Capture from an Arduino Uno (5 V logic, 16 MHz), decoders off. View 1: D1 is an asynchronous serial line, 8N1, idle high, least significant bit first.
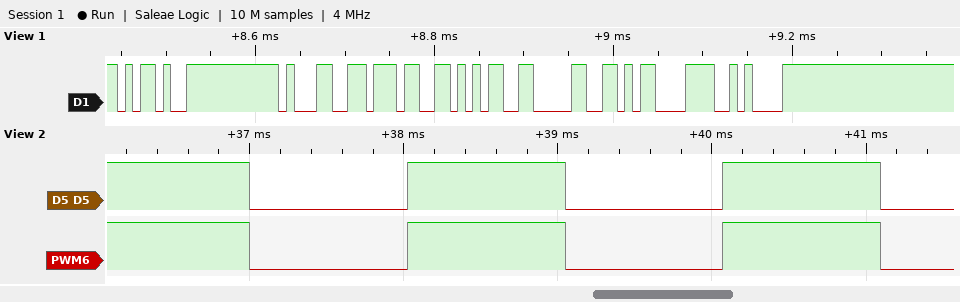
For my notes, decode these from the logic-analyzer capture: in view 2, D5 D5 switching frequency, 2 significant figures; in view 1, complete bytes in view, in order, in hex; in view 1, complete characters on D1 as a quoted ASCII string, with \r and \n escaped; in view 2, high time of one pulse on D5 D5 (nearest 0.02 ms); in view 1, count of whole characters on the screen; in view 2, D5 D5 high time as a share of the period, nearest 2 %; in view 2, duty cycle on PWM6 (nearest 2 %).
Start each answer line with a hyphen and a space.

- 490 Hz
- 0x2D 0x31 0x37 0x35 0x30 0x0D 0x0A
- "-1750\r\n"
- 1.02 ms
- 7
- 50 %
- 50 %
